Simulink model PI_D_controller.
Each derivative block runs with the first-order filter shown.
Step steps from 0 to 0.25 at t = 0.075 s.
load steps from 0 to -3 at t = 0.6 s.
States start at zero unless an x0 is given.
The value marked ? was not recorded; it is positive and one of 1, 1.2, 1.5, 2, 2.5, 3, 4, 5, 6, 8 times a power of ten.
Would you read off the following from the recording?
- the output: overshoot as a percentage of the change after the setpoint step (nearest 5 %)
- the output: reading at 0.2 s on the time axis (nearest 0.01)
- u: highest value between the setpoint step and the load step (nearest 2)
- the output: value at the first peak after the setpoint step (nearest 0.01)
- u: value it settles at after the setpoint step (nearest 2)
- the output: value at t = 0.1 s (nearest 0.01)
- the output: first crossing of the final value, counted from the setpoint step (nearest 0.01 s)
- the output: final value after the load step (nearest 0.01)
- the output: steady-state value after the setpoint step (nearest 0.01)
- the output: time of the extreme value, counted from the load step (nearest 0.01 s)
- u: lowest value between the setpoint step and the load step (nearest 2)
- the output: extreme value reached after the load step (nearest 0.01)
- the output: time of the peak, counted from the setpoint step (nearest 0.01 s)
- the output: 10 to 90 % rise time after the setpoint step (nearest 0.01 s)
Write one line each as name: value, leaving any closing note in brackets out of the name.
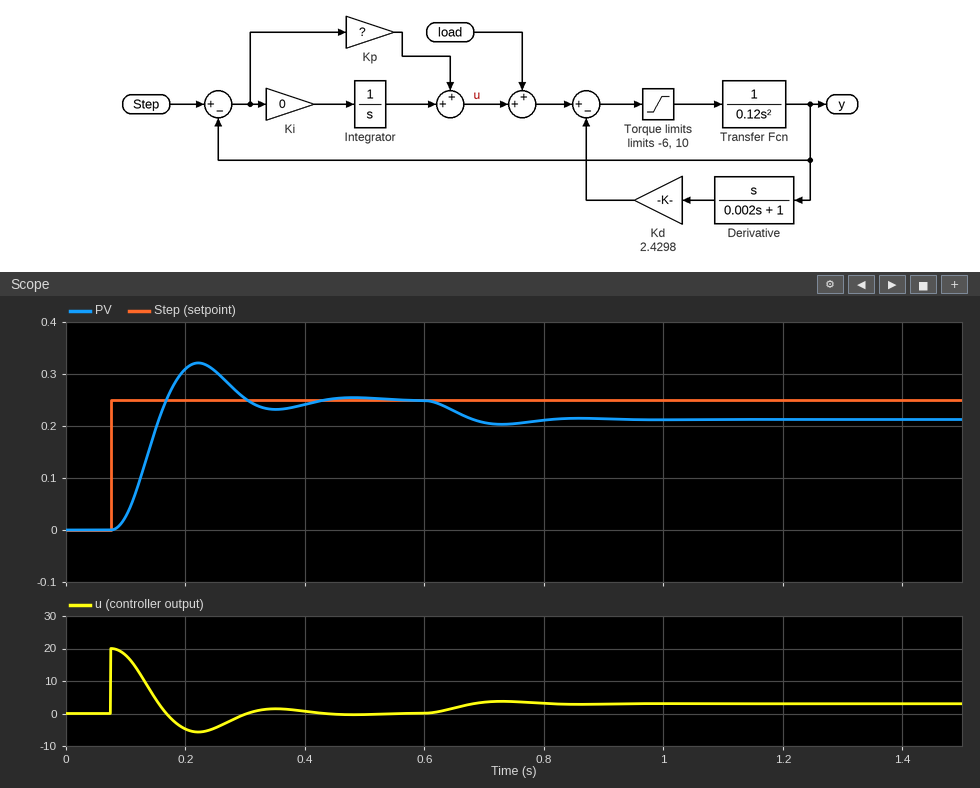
the output: overshoot as a percentage of the change after the setpoint step: 30 %
the output: reading at 0.2 s on the time axis: 0.31
u: highest value between the setpoint step and the load step: 20
the output: value at the first peak after the setpoint step: 0.32
u: value it settles at after the setpoint step: 0
the output: value at t = 0.1 s: 0.03
the output: first crossing of the final value, counted from the setpoint step: 0.09 s
the output: final value after the load step: 0.21
the output: steady-state value after the setpoint step: 0.25
the output: time of the extreme value, counted from the load step: 0.13 s
u: lowest value between the setpoint step and the load step: -6
the output: extreme value reached after the load step: 0.20
the output: time of the peak, counted from the setpoint step: 0.15 s
the output: 10 to 90 % rise time after the setpoint step: 0.06 s
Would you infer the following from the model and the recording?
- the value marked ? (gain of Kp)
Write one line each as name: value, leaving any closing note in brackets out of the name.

the value marked ?: 80
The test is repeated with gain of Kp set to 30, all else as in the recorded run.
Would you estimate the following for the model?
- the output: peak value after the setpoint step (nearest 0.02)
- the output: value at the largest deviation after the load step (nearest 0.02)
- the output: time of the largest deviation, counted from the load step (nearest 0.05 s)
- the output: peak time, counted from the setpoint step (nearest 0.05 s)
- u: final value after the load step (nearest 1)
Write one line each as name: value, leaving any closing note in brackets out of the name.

the output: peak value after the setpoint step: 0.26
the output: value at the largest deviation after the load step: 0.14
the output: time of the largest deviation, counted from the load step: 0.25 s
the output: peak time, counted from the setpoint step: 0.25 s
u: final value after the load step: 3
